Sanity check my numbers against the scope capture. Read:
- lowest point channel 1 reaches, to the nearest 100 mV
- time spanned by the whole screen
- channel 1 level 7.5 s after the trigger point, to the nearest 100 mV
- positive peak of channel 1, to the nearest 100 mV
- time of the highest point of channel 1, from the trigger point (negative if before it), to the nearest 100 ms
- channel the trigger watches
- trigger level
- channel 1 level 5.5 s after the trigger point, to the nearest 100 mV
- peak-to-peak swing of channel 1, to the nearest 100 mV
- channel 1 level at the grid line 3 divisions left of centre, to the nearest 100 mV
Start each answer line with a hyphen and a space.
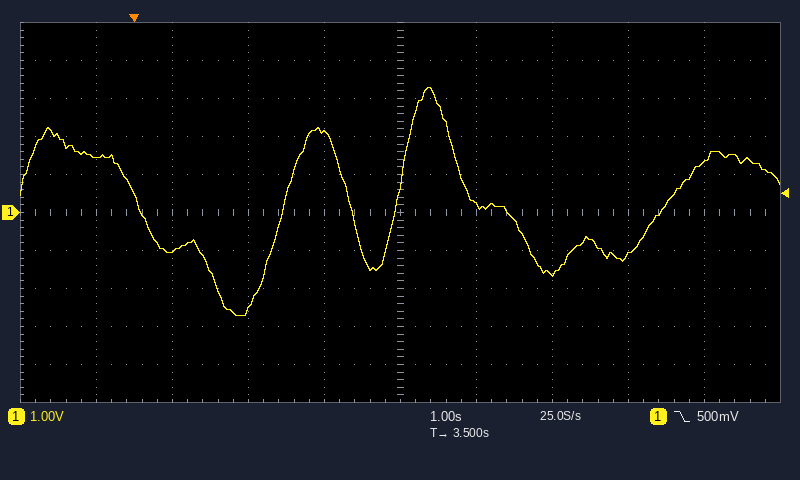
- -2.7 V
- 10 s
- 1.3 V
- 3.3 V
- +3.9 s
- channel 1
- 500 mV
- -1.6 V
- 6.0 V
- -1.0 V
